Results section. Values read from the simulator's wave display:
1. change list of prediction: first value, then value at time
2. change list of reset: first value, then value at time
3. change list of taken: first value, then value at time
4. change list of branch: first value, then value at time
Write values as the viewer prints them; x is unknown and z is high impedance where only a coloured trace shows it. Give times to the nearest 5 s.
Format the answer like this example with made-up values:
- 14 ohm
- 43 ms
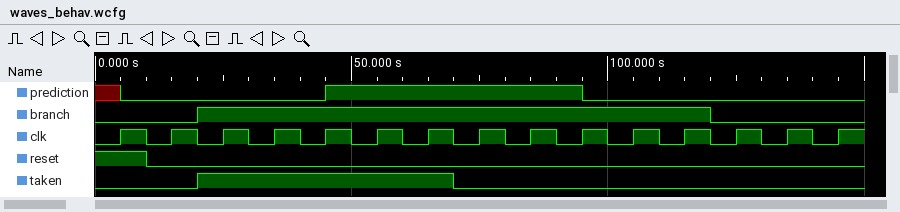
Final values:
- x, 0 at 5 s, 1 at 45 s, 0 at 95 s
- 1, 0 at 10 s
- 0, 1 at 20 s, 0 at 70 s
- 0, 1 at 20 s, 0 at 120 s
